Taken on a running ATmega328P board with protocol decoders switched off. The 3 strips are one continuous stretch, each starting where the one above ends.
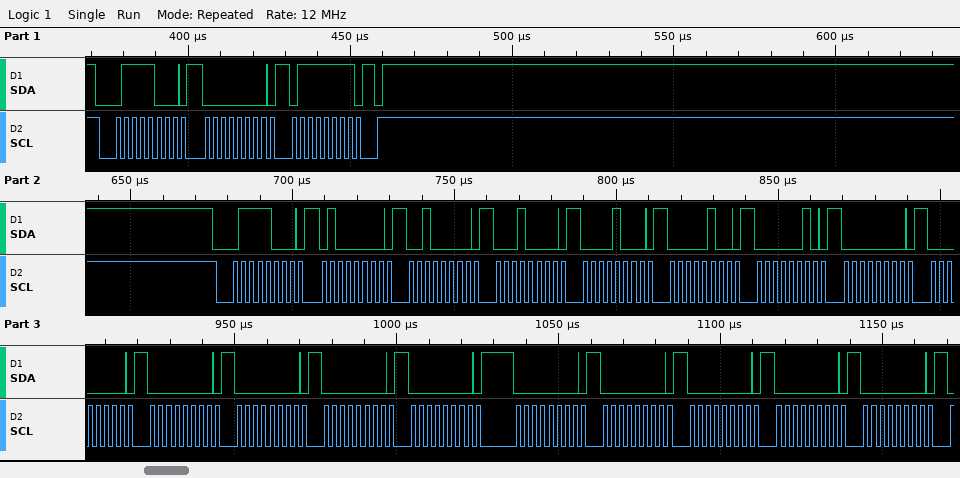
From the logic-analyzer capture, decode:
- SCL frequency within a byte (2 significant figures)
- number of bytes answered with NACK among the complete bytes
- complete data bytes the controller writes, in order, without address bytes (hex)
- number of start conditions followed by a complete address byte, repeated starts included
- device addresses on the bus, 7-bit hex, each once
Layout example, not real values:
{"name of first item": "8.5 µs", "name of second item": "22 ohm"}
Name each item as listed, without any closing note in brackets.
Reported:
{"SCL frequency within a byte": "400 kHz", "number of bytes answered with NACK among the complete bytes": "0", "complete data bytes the controller writes, in order, without address bytes": "00 7F 40 20 10 08 04 02 00 00 00 00 00 00 00 00 00 00 00", "number of start conditions followed by a complete address byte, repeated starts included": "2", "device addresses on the bus, 7-bit hex, each once": "0x3C"}
